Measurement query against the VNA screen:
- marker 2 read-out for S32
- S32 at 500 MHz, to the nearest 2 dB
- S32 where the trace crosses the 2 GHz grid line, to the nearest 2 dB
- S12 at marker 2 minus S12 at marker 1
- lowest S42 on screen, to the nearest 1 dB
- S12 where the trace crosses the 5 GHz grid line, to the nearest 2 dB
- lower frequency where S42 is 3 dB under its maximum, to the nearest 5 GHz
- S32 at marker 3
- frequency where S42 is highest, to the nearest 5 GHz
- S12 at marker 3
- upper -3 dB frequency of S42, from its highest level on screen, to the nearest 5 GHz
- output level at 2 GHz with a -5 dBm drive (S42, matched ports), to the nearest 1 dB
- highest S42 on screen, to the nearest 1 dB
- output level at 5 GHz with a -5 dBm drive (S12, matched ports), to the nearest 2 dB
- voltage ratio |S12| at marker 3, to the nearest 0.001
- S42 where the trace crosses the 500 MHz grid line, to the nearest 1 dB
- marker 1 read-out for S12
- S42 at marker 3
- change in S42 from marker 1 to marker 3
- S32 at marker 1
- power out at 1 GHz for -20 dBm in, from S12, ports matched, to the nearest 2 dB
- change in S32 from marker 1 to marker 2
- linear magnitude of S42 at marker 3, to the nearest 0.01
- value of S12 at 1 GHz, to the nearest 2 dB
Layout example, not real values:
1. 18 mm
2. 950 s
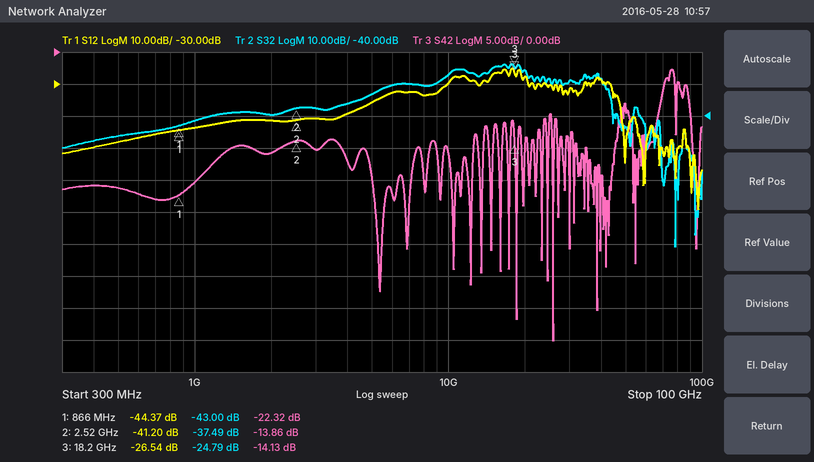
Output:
1. -37.49 dB
2. -46 dB
3. -40 dB
4. 3.17 dB
5. -45 dB
6. -36 dB
7. 70 GHz
8. -24.79 dB
9. 75 GHz
10. -26.54 dB
11. 80 GHz
12. -21 dBm
13. -3 dB
14. -40 dBm
15. 0.047
16. -21 dB
17. -44.37 dB
18. -14.13 dB
19. 8.19 dB
20. -43.00 dB
21. -64 dBm
22. 5.51 dB
23. 0.20
24. -44 dB
